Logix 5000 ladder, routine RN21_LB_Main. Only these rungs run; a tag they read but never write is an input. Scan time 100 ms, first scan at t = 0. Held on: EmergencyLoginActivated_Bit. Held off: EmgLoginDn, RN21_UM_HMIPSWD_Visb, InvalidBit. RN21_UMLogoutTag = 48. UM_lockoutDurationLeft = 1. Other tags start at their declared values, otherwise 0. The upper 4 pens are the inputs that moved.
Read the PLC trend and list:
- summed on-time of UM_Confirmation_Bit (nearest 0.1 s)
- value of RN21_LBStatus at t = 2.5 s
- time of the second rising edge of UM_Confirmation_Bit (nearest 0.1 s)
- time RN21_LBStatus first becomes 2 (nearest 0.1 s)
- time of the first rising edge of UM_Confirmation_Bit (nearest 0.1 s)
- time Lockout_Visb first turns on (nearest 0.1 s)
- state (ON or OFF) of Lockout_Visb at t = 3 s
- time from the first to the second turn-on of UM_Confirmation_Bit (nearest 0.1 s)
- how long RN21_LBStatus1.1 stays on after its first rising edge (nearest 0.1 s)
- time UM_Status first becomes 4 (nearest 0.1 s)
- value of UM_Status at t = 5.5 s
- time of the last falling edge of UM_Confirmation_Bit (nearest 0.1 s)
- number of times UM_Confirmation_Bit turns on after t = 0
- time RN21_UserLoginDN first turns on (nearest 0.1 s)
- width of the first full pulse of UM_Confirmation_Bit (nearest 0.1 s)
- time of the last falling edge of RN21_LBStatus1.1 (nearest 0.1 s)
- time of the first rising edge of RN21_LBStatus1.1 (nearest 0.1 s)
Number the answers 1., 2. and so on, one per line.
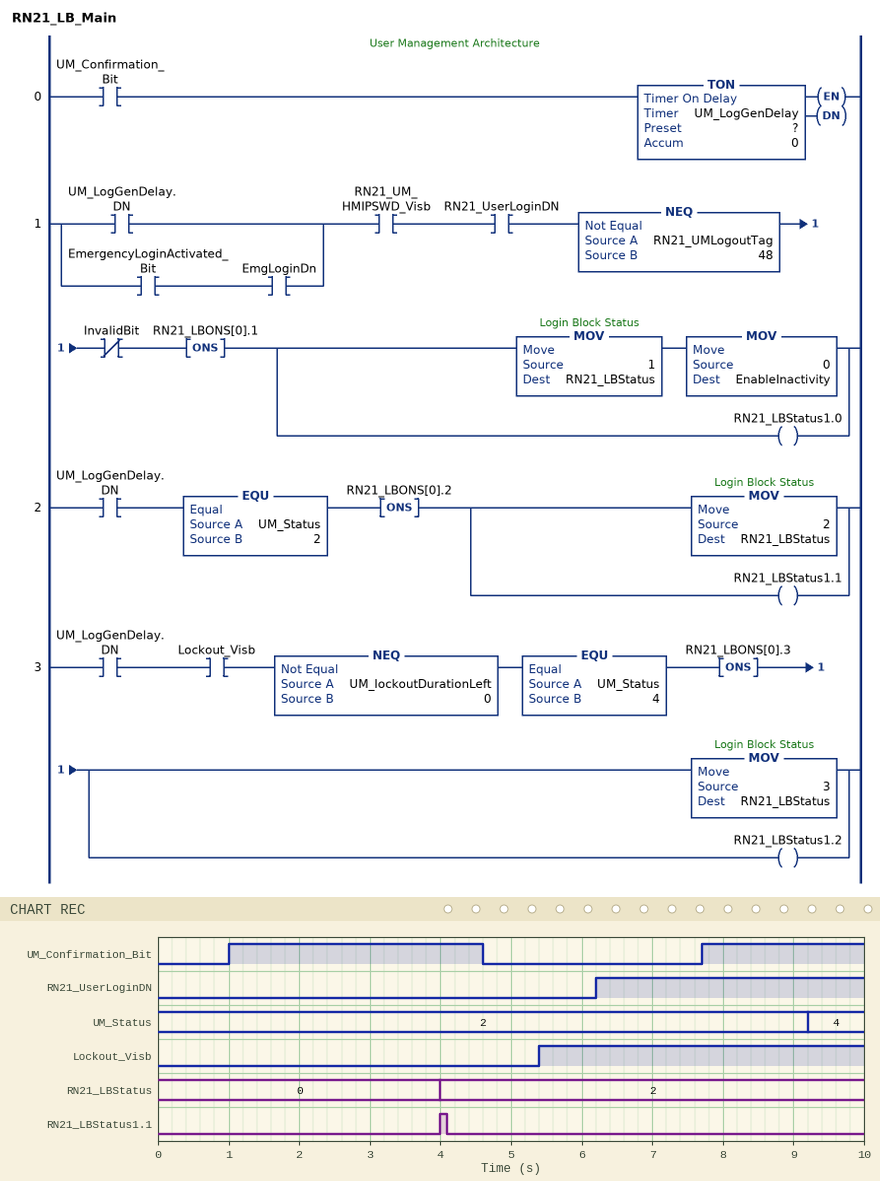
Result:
1. 5.9 s
2. 0
3. 7.7 s
4. 4.0 s
5. 1.0 s
6. 5.4 s
7. OFF
8. 6.7 s
9. 0.1 s
10. 9.2 s
11. 2
12. 4.6 s
13. 2
14. 6.2 s
15. 3.6 s
16. 4.1 s
17. 4.0 s
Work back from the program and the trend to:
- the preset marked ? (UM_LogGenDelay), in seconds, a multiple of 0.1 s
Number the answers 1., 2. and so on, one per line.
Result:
1. 3.0 s
